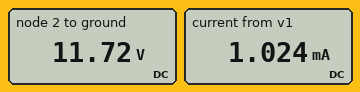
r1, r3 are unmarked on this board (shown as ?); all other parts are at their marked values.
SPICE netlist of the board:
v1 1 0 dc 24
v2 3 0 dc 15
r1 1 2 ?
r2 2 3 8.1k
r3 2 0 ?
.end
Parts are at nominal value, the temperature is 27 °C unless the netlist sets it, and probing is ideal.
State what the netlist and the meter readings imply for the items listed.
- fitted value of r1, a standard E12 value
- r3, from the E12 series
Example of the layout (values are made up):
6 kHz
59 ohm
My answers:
12 kΩ
8.2 kΩ
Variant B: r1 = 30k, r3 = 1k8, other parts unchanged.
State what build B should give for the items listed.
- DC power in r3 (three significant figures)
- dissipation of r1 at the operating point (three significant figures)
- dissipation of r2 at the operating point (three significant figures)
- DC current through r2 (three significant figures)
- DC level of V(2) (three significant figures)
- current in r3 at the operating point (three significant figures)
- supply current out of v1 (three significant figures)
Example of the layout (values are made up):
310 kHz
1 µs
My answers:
7.70 mW
13.7 mW
15.7 mW
1.39 mA
3.72 V
2.07 mA
676 µA
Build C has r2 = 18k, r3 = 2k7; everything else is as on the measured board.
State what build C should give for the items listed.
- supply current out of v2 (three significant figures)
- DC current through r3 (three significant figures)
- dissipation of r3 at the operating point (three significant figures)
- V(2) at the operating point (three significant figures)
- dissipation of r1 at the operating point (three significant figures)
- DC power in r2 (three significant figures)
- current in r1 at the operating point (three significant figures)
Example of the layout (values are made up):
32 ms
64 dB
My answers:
524 µA
2.06 mA
11.5 mW
5.56 V
28.3 mW
4.95 mW
1.54 mA
